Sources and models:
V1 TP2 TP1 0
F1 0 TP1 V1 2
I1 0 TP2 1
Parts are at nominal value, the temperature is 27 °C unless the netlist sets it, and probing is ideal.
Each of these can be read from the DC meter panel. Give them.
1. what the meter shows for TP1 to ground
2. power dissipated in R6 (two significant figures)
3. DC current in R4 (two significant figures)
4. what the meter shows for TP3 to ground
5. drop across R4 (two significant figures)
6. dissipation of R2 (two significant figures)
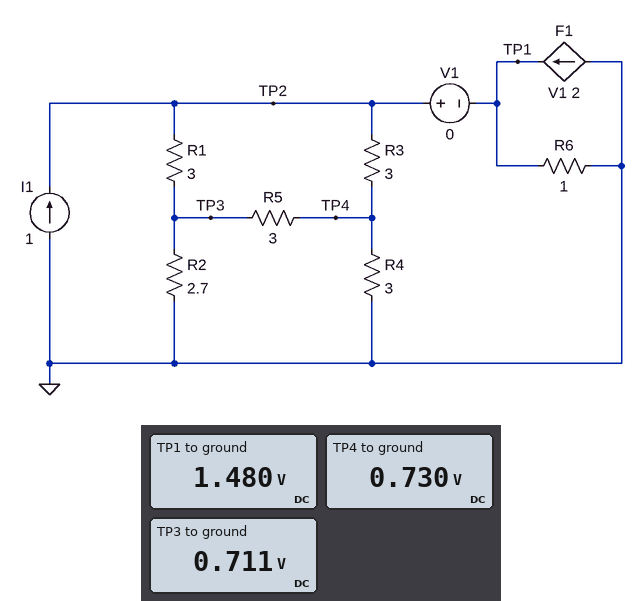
1.480 V
2.2 W
240 mA
0.711 V
730 mV
190 mW
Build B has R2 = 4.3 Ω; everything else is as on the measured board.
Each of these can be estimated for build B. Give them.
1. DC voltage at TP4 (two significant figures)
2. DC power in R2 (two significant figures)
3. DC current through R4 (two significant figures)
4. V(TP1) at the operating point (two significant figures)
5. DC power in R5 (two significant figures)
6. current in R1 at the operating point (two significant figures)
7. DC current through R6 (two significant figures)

820 mV
180 mW
270 mA
1.6 V
1.5 mW
230 mA
1.6 A
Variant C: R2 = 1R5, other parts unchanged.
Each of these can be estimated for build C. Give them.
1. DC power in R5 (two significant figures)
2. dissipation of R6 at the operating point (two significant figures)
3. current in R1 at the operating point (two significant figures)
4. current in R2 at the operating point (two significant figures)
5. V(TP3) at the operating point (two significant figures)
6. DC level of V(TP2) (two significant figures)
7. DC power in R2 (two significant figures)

5.2 mW
1.9 W
290 mA
330 mA
500 mV
1.4 V
170 mW
